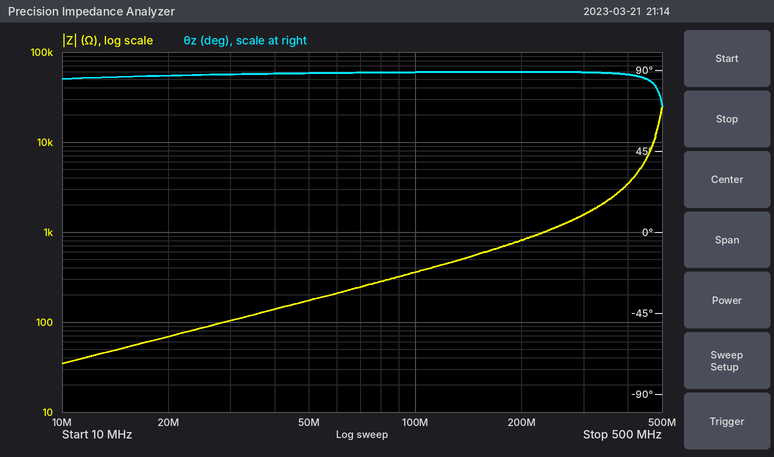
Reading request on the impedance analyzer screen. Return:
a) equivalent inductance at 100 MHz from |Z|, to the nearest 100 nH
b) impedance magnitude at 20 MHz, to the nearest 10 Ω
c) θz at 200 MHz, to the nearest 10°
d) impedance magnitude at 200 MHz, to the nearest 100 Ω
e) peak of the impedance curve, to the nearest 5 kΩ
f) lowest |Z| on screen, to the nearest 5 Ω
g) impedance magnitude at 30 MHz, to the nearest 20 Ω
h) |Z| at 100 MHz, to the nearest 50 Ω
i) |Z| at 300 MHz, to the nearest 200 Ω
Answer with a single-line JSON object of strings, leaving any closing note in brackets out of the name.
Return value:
{"equivalent inductance at 100 MHz from |Z|, to the nearest 100 nH": "600 nH", "impedance magnitude at 20 MHz, to the nearest 10 Ω": "70 Ω", "θz at 200 MHz, to the nearest 10°": "90°", "impedance magnitude at 200 MHz, to the nearest 100 Ω": "800 Ω", "peak of the impedance curve, to the nearest 5 kΩ": "25 kΩ", "lowest |Z| on screen, to the nearest 5 Ω": "35 Ω", "impedance magnitude at 30 MHz, to the nearest 20 Ω": "100 Ω", "|Z| at 100 MHz, to the nearest 50 Ω": "350 Ω", "|Z| at 300 MHz, to the nearest 200 Ω": "1.6 kΩ"}
